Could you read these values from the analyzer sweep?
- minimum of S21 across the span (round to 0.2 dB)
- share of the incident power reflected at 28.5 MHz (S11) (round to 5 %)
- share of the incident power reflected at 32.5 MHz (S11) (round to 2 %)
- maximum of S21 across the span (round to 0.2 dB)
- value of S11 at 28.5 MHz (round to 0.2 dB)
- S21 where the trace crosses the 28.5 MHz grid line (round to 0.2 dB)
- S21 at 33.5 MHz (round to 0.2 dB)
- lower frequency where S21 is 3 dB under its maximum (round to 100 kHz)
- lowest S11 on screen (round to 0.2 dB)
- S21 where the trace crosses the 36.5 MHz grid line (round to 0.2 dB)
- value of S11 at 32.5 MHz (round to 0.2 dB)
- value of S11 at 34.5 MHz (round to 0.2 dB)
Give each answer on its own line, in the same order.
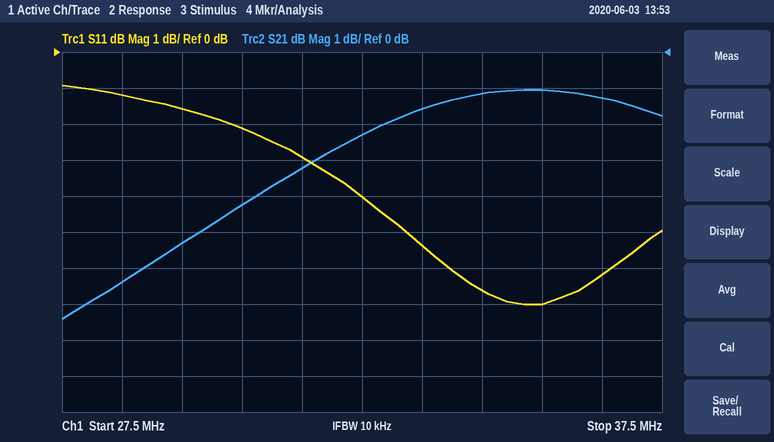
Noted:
-7.4 dB
75 %
40 %
-1.0 dB
-1.2 dB
-6.4 dB
-1.6 dB
30.7 MHz
-7.0 dB
-1.2 dB
-4.0 dB
-6.6 dB
